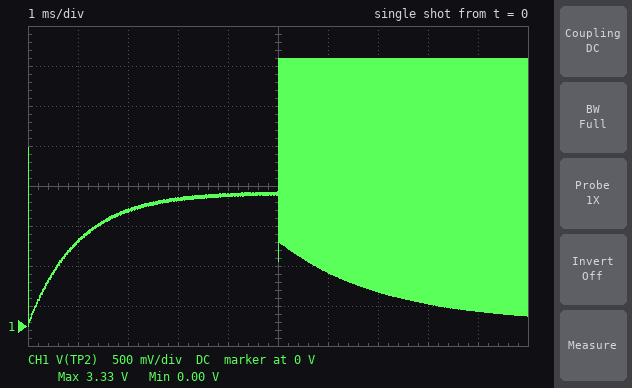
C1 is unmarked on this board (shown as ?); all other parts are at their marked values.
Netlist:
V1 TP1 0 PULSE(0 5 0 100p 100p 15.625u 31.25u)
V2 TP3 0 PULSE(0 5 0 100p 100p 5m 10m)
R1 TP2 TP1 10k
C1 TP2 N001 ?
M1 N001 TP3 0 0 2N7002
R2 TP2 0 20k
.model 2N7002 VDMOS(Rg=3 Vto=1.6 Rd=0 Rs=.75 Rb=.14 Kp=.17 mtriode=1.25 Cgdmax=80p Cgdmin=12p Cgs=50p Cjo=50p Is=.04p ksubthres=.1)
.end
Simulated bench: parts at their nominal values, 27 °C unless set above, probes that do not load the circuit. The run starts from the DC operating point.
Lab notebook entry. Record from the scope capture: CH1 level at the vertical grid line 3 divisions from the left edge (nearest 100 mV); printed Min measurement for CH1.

1.6 V
0.00 V
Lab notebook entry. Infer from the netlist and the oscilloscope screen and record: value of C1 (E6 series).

150 nF
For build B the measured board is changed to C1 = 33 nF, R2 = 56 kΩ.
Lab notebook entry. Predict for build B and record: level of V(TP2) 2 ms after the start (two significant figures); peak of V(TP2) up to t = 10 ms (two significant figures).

2.1 V
4.2 V
